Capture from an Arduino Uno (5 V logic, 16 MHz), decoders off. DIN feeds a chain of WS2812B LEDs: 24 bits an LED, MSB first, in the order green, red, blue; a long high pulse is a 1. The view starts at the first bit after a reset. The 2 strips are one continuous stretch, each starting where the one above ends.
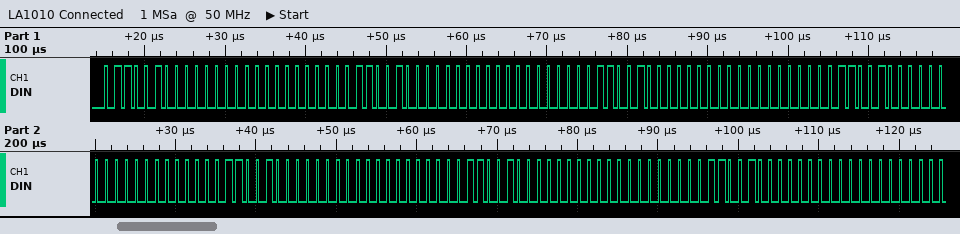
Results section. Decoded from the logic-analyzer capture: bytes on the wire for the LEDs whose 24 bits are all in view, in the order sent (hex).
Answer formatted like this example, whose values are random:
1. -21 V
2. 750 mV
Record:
1. 64 00 00 64 00 00 64 00 00 64 00 00 64 00 00 64 00 00 64 00 00
